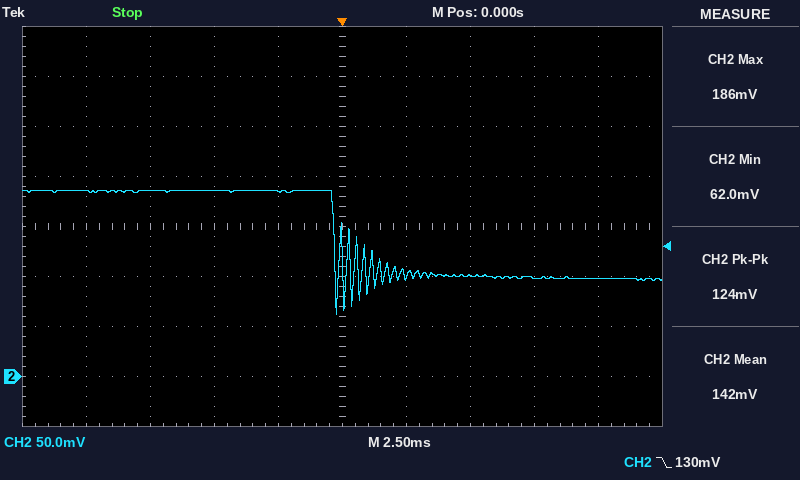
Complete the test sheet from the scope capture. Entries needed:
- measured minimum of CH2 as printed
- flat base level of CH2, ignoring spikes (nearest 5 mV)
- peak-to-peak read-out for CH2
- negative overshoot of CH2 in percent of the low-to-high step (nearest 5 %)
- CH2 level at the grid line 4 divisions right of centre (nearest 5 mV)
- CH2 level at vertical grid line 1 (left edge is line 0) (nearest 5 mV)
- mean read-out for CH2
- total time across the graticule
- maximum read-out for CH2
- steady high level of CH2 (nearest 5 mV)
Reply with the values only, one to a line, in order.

62.0 mV
100 mV
124 mV
40 %
100 mV
185 mV
142 mV
25 ms
186 mV
185 mV
